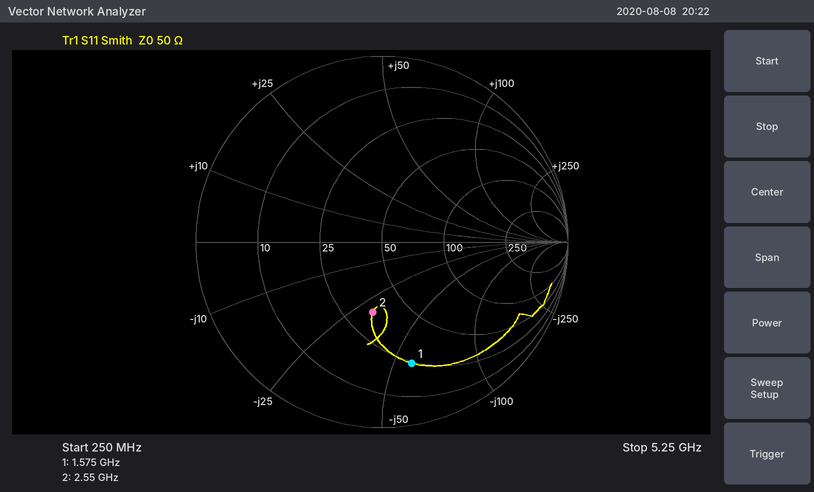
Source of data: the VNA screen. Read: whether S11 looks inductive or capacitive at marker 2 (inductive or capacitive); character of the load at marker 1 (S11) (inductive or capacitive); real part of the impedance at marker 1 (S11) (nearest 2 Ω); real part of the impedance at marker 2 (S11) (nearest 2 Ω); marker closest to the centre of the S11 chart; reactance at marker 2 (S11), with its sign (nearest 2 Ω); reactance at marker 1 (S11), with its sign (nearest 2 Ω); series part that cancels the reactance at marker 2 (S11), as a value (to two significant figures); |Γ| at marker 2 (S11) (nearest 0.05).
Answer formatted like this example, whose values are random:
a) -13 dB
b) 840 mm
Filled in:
a) capacitive
b) capacitive
c) 24 Ω
d) 34 Ω
e) marker 2
f) -30 Ω
g) -58 Ω
h) 1.9 nH
i) 0.40
